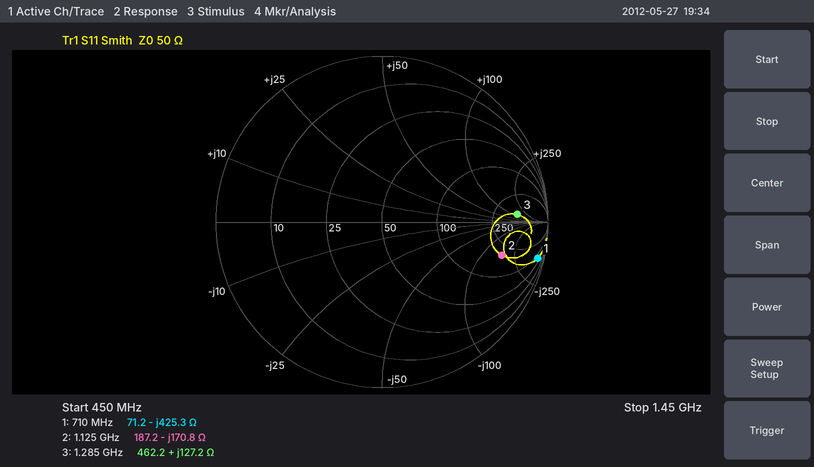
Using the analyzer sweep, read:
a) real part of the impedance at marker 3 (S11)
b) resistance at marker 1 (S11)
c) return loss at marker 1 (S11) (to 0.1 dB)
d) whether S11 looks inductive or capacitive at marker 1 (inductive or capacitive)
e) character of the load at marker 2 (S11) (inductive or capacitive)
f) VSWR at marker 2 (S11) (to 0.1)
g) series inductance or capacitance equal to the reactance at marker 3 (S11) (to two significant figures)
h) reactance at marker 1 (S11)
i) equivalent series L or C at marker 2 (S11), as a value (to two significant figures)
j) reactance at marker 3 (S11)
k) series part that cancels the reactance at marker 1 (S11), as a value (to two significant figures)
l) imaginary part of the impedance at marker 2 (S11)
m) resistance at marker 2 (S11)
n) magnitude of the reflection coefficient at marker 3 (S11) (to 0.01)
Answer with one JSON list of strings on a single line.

["462.2 Ω", "71.2 Ω", "0.3 dB", "capacitive", "capacitive", "7.0", "16 nH", "-425.3 Ω", "830 fF", "+127.2 Ω", "95 nH", "-170.8 Ω", "187.2 Ω", "0.82"]
